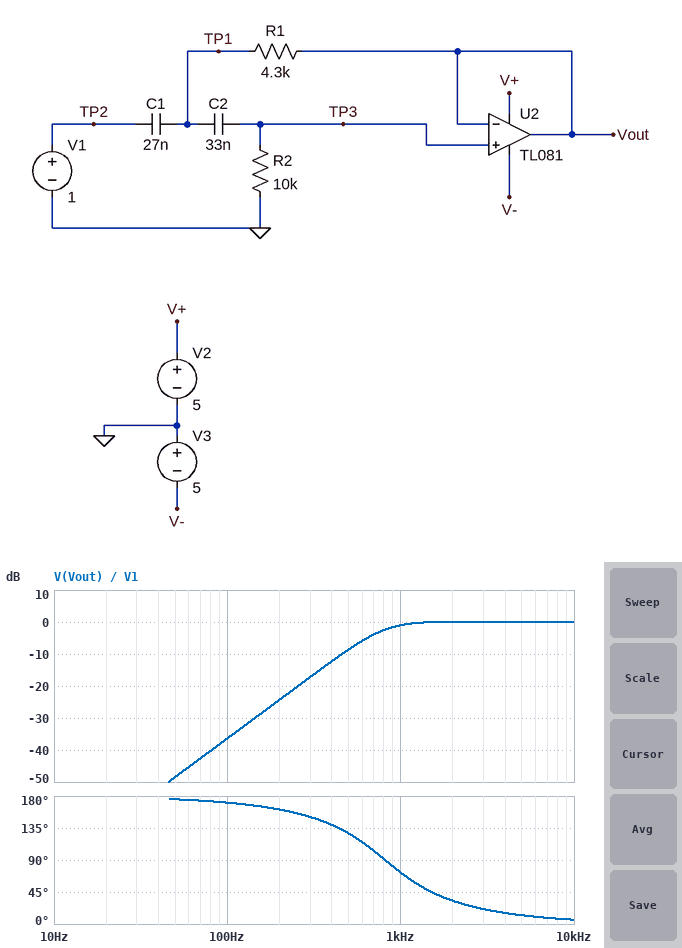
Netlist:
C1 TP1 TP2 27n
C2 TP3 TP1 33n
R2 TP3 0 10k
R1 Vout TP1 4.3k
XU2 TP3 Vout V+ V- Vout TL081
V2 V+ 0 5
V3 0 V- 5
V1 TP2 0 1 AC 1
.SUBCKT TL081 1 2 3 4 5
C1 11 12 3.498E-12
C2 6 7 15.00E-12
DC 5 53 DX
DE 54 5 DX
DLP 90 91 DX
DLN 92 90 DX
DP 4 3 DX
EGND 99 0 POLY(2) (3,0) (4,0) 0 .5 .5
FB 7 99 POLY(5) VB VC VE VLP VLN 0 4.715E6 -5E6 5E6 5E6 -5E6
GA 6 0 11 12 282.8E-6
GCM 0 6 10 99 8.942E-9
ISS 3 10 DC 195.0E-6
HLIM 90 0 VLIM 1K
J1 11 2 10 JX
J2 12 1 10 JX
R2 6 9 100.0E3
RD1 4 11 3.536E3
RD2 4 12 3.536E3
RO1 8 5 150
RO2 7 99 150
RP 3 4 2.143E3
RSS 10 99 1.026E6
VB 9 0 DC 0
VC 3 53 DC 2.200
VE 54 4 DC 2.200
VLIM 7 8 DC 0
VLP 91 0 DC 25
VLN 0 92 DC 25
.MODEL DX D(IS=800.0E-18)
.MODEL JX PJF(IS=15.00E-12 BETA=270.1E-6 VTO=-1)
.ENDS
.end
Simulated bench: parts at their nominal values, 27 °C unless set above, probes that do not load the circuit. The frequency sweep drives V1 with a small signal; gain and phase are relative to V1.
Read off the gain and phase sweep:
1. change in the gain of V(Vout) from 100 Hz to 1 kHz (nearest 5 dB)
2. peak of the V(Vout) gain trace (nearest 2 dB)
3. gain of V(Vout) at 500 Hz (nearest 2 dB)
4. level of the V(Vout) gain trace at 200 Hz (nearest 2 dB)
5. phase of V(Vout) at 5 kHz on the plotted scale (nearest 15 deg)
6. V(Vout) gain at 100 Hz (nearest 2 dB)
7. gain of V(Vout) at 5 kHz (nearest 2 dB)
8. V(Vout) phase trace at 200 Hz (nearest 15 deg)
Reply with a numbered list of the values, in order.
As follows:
1. 35 dB
2. 0 dB
3. -8 dB
4. -24 dB
5. 15 deg
6. -36 dB
7. 0 dB
8. 165 deg
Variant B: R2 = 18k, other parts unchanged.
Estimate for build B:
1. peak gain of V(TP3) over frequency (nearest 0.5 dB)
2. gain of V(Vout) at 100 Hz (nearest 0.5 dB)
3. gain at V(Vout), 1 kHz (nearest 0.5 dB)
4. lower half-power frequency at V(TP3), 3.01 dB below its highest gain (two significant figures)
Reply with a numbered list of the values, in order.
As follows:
1. 1.5 dB
2. -31.0 dB
3. 1.0 dB
4. 520 Hz
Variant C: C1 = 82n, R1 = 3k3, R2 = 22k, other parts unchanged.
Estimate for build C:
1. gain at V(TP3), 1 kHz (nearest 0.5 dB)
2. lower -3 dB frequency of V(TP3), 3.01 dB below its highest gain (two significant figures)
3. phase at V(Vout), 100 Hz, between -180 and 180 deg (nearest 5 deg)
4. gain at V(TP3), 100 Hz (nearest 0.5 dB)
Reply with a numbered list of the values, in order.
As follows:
1. 0.5 dB
2. 300 Hz
3. 165 deg
4. -22.0 dB
